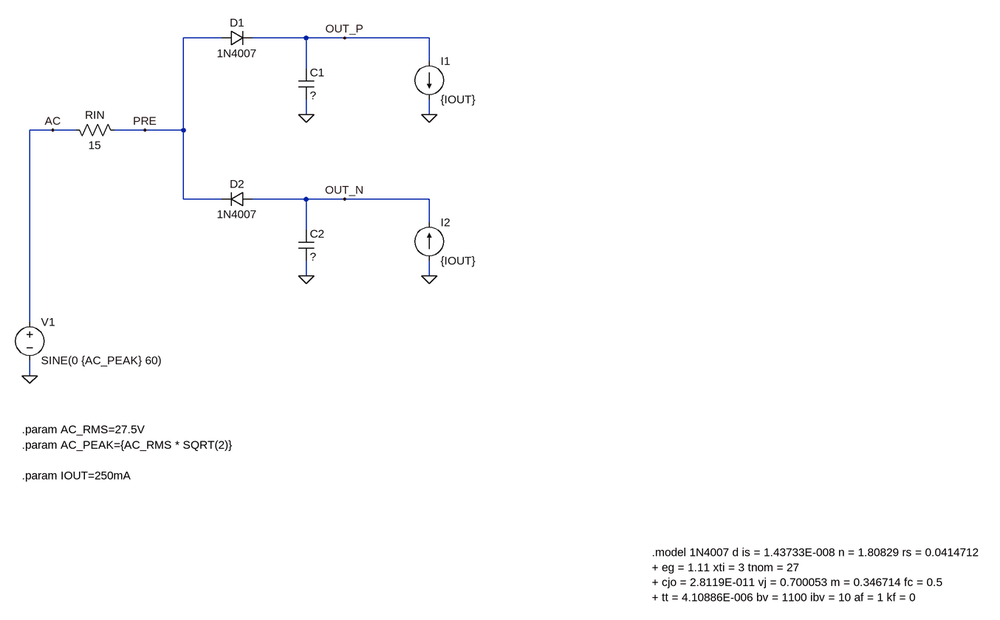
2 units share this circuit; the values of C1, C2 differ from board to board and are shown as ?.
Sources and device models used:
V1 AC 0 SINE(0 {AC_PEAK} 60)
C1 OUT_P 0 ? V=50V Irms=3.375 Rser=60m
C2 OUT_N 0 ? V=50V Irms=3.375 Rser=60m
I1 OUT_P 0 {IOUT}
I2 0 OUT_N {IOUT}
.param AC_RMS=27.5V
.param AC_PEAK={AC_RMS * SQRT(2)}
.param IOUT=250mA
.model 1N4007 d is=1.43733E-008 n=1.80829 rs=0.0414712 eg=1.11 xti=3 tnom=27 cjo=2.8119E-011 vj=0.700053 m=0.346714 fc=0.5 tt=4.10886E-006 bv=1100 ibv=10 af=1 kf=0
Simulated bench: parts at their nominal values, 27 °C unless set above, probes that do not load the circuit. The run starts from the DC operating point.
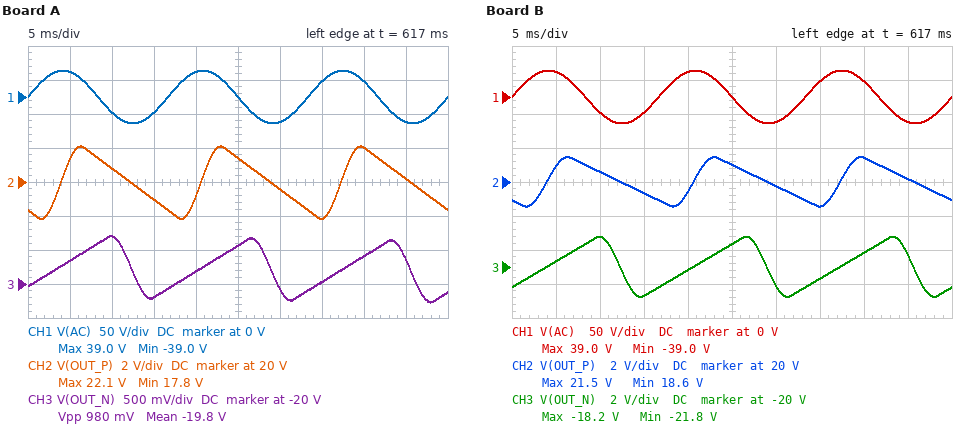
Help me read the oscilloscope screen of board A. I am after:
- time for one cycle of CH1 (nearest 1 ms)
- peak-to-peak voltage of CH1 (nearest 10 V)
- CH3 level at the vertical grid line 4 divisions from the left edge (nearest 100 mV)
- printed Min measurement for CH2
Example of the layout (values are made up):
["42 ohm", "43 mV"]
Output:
["17 ms", "80 V", "-19.8 V", "17.8 V"]
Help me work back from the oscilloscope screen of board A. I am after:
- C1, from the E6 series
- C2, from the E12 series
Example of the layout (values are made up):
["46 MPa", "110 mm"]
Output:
["680 µF", "3.3 mF"]
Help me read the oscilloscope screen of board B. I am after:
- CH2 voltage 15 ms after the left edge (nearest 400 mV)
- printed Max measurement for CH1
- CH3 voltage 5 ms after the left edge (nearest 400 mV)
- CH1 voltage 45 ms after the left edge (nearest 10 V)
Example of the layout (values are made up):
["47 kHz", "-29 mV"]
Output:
["19.2 V", "39.0 V", "-19.6 V", "-40 V"]
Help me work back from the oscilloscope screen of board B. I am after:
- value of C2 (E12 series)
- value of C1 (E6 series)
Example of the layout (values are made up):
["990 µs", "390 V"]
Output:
["820 µF", "1 mF"]
